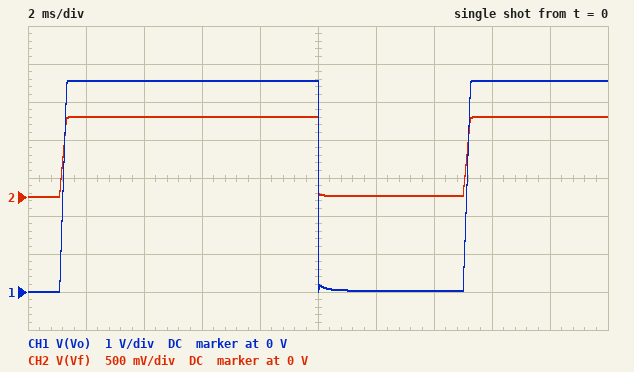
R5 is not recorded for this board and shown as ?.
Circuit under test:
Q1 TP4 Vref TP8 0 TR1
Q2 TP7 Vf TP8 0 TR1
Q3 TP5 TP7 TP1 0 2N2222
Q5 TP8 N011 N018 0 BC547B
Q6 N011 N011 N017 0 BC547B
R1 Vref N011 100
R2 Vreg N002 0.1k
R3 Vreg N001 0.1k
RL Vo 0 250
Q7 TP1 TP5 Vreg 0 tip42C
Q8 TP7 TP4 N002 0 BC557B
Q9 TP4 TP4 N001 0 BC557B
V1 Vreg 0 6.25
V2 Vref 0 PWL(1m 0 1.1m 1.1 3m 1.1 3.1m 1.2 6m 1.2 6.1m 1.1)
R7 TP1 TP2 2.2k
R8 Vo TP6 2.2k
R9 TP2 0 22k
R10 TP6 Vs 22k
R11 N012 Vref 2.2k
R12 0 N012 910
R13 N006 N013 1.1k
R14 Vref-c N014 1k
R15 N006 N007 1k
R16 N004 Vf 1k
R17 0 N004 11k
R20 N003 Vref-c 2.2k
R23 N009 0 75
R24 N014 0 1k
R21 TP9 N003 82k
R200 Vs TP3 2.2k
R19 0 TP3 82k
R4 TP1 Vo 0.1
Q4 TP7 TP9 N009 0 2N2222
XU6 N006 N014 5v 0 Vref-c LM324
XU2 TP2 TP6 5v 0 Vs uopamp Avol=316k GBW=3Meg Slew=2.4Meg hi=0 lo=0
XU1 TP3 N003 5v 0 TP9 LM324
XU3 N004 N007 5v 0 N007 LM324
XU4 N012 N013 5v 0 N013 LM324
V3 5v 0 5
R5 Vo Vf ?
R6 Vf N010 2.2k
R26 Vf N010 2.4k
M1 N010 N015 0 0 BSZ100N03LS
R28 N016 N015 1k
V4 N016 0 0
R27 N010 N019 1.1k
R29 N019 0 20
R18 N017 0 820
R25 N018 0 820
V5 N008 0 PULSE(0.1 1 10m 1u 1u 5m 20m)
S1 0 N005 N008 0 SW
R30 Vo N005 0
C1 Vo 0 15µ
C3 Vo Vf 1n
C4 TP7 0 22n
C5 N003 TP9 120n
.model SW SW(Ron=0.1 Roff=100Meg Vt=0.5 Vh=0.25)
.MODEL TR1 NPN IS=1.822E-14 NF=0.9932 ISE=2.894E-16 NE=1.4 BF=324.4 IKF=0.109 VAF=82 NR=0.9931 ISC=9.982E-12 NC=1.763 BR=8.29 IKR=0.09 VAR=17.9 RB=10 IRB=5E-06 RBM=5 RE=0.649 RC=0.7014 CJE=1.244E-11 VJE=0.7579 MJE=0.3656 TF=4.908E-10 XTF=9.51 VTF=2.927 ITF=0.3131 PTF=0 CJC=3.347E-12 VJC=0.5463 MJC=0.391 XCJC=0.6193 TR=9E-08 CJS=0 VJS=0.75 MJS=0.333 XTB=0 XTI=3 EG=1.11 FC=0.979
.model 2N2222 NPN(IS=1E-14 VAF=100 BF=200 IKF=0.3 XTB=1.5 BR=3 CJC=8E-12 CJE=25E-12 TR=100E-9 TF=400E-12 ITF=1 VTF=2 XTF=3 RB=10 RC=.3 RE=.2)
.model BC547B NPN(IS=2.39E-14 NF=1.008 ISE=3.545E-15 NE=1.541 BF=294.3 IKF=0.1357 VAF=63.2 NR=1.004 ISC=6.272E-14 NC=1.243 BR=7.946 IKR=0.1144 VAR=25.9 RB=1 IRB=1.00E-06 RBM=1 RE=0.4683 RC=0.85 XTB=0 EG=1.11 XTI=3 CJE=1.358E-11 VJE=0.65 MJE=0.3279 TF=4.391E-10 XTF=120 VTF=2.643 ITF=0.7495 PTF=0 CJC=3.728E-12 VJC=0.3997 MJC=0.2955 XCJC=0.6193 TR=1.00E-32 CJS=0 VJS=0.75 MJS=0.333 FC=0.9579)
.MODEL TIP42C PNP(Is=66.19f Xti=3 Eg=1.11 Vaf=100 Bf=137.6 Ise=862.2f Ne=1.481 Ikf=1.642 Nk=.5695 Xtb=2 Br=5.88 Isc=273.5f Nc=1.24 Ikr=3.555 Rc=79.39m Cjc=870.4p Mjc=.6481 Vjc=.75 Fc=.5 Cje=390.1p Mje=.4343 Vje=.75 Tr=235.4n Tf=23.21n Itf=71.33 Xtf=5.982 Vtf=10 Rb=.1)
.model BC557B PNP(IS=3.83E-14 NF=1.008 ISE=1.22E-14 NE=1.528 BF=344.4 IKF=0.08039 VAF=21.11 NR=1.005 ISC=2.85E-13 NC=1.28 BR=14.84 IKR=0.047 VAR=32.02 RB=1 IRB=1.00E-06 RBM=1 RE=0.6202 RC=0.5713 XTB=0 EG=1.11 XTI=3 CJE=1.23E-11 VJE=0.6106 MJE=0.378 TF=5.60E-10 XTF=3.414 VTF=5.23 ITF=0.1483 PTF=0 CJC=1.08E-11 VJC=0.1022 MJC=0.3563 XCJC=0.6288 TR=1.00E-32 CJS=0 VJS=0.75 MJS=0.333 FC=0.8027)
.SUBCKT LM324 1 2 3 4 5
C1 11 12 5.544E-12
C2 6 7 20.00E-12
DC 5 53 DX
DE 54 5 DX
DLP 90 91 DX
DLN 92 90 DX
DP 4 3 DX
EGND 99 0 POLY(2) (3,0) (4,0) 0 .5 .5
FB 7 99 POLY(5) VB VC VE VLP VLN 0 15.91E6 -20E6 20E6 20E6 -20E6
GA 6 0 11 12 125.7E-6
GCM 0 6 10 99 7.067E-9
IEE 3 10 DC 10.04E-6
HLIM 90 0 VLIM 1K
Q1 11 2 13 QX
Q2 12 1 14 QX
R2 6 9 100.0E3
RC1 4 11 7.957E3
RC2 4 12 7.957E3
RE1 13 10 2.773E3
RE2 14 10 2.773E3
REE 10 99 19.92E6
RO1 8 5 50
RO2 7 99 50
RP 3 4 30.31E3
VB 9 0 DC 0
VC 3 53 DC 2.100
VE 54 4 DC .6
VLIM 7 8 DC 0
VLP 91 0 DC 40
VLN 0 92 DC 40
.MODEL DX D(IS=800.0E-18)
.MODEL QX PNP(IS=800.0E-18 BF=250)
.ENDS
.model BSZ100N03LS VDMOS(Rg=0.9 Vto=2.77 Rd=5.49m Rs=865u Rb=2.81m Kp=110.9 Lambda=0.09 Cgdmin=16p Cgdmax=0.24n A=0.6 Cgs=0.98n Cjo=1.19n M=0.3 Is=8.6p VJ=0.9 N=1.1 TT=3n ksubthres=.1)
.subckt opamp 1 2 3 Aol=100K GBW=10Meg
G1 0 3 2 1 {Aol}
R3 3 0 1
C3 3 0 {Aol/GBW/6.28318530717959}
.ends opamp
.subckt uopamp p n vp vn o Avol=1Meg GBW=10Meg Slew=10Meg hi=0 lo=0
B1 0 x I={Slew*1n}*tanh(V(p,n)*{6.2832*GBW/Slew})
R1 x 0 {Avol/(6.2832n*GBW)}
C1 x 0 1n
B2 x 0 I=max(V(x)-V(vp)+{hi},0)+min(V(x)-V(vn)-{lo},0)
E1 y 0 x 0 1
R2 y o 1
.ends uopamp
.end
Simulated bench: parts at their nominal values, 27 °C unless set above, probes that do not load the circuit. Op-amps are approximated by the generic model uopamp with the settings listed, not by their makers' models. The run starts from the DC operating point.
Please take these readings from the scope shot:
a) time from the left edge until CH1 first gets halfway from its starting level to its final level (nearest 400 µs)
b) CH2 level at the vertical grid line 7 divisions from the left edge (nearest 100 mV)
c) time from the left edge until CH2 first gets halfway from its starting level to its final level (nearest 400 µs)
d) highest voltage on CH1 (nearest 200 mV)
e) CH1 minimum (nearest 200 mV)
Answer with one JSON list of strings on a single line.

["1.2 ms", "0 V", "1.2 ms", "5.6 V", "0 V"]
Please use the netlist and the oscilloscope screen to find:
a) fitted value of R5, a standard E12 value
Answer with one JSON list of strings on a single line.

["8.2 kΩ"]
